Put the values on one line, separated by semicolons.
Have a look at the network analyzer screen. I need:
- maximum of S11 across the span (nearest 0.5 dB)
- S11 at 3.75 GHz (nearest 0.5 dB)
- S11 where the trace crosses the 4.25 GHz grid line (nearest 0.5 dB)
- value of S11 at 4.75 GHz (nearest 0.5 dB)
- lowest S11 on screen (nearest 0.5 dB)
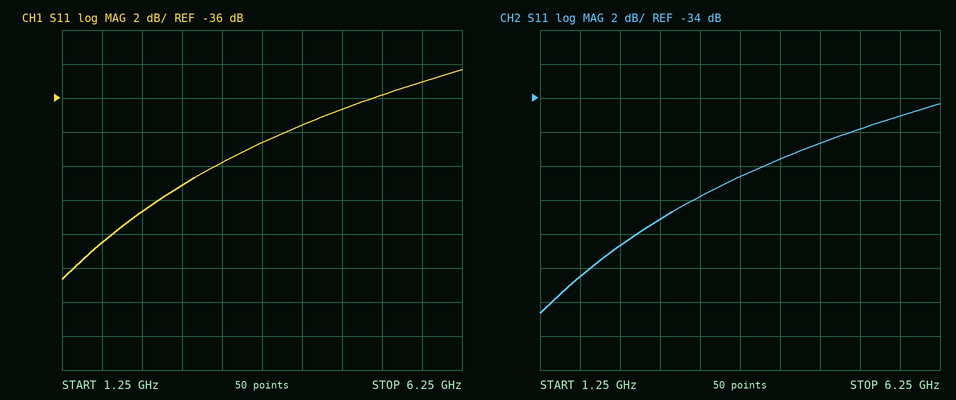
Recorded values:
-34.5 dB; -38.5 dB; -37.5 dB; -36.5 dB; -46.5 dB
